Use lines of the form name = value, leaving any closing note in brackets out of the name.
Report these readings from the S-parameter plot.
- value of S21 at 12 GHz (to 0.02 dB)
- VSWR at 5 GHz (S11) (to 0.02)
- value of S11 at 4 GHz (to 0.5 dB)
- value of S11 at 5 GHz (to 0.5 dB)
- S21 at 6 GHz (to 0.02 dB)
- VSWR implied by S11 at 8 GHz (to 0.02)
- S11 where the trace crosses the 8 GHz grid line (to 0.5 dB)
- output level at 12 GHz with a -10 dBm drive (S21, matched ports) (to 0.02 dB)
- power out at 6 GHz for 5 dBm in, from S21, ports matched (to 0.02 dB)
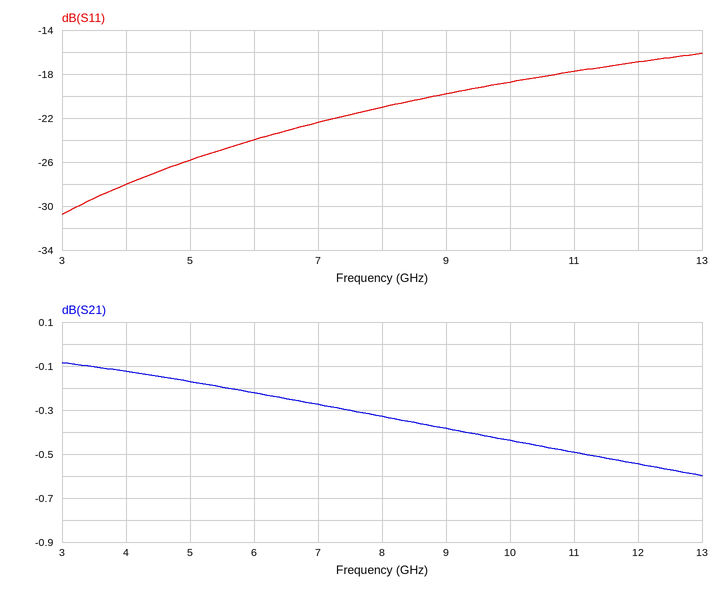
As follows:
value of S21 at 12 GHz = -0.54 dB
VSWR at 5 GHz (S11) = 1.10
value of S11 at 4 GHz = -28.0 dB
value of S11 at 5 GHz = -26.0 dB
S21 at 6 GHz = -0.22 dB
VSWR implied by S11 at 8 GHz = 1.20
S11 where the trace crosses the 8 GHz grid line = -21.0 dB
output level at 12 GHz with a -10 dBm drive (S21, matched ports) = -10.54 dBm
power out at 6 GHz for 5 dBm in, from S21, ports matched = 4.78 dBm
